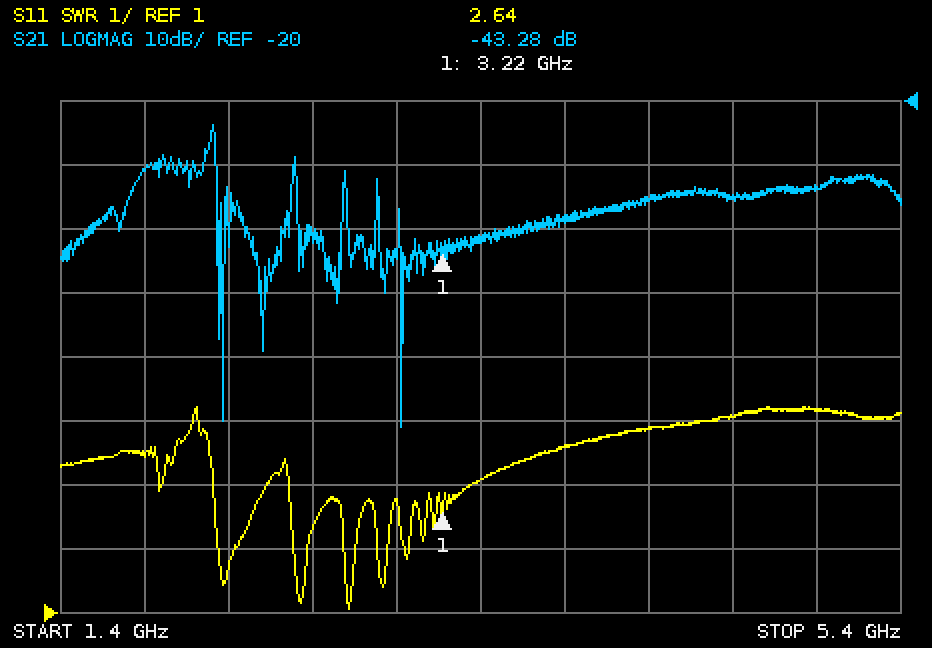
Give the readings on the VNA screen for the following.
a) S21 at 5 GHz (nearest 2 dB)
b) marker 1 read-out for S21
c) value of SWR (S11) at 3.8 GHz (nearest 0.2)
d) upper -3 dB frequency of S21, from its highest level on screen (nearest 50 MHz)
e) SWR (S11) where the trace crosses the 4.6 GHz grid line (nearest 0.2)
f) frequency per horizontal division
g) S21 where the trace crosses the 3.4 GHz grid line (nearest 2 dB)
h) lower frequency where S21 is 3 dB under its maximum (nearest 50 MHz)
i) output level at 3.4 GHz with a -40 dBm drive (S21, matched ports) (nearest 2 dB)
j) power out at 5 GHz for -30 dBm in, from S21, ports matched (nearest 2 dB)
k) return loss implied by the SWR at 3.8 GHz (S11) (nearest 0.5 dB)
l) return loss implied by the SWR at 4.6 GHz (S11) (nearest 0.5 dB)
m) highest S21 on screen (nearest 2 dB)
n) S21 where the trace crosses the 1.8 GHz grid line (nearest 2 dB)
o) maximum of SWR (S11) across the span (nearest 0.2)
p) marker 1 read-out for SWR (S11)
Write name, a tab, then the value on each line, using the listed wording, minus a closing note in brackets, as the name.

S21 at 5 GHz	-34 dB
marker 1 read-out for S21	-43.28 dB
value of SWR (S11) at 3.8 GHz	3.6
upper -3 dB frequency of S21, from its highest level on screen	2.15 GHz
SWR (S11) where the trace crosses the 4.6 GHz grid line	4.0
frequency per horizontal division	400 MHz
S21 where the trace crosses the 3.4 GHz grid line	-42 dB
lower frequency where S21 is 3 dB under its maximum	2.10 GHz
output level at 3.4 GHz with a -40 dBm drive (S21, matched ports)	-82 dBm
power out at 5 GHz for -30 dBm in, from S21, ports matched	-64 dBm
return loss implied by the SWR at 3.8 GHz (S11)	5.0 dB
return loss implied by the SWR at 4.6 GHz (S11)	4.5 dB
highest S21 on screen	-24 dB
S21 where the trace crosses the 1.8 GHz grid line	-30 dB
maximum of SWR (S11) across the span	4.2
marker 1 read-out for SWR	2.64
